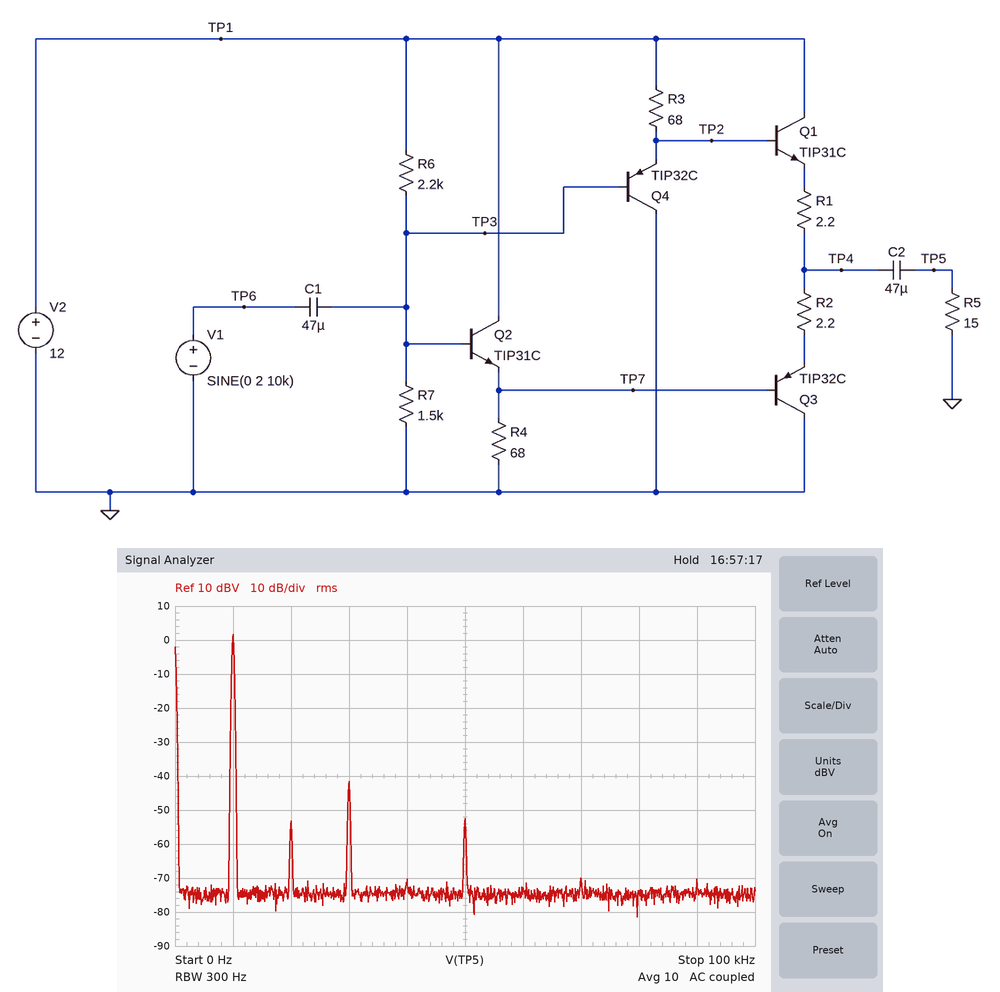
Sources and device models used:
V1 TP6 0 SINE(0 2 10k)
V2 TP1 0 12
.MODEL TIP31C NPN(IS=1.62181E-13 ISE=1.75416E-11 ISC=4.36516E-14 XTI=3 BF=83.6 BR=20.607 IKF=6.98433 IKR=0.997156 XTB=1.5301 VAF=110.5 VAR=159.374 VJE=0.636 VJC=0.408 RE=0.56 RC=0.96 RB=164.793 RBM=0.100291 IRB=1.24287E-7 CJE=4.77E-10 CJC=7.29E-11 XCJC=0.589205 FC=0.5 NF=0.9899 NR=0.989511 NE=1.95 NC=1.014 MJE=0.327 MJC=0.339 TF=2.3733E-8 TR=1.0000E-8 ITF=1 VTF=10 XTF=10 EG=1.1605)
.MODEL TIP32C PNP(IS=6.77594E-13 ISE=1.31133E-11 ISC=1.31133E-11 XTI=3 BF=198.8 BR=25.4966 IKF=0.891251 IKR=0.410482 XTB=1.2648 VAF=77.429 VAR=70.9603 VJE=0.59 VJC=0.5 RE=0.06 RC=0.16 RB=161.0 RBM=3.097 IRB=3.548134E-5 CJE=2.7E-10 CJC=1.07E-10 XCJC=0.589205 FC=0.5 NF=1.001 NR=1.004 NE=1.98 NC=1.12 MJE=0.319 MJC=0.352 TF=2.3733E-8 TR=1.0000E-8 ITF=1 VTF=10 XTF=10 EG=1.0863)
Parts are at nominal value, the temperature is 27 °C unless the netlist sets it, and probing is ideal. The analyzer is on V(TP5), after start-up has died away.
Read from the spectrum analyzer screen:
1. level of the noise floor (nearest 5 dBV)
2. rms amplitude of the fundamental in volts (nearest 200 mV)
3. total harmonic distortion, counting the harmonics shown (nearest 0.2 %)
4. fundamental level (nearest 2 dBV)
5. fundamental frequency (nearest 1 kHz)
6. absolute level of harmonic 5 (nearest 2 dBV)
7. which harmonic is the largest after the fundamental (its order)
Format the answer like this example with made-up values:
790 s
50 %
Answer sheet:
-75 dBV
1.2 V
0.8 %
2 dBV
10 kHz
-52 dBV
3
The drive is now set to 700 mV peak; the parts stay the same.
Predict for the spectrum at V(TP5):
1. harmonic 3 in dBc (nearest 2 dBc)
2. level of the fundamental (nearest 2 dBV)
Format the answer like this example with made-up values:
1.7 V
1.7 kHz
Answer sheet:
-56 dBc
-8 dBV
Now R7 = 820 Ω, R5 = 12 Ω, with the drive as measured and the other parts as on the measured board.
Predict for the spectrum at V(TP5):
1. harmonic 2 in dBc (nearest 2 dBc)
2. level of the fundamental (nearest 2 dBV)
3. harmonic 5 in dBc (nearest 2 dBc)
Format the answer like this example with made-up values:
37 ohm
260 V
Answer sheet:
-60 dBc
2 dBV
-50 dBc
